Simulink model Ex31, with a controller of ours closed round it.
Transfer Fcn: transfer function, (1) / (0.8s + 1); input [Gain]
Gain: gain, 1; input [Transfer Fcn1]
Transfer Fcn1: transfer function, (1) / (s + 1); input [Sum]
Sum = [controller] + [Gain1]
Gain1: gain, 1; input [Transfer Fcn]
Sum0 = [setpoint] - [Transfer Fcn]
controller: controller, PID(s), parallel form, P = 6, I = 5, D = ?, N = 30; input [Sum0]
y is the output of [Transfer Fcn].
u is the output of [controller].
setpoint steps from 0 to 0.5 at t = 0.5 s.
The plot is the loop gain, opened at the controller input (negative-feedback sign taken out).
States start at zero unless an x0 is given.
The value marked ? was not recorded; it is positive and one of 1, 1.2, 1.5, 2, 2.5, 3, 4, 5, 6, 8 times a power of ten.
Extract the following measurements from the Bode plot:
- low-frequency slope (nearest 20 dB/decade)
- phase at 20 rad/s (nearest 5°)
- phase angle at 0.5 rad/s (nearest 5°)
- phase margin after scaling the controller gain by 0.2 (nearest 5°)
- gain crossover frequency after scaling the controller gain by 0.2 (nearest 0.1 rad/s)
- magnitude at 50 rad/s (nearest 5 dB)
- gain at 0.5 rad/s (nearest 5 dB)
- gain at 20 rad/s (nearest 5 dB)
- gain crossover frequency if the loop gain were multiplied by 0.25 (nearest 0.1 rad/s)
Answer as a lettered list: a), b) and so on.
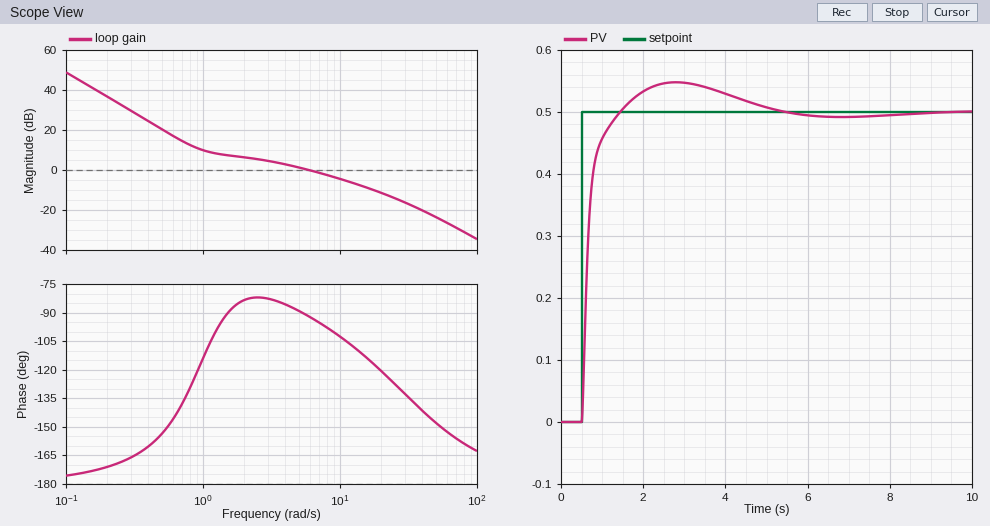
a) -40 dB/decade
b) -120°
c) -155°
d) 45°
e) 0.7 rad/s
f) -25 dB
g) 20 dB
h) -10 dB
i) 0.8 rad/s
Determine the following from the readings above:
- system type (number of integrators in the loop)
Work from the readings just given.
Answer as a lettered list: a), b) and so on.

a) 2
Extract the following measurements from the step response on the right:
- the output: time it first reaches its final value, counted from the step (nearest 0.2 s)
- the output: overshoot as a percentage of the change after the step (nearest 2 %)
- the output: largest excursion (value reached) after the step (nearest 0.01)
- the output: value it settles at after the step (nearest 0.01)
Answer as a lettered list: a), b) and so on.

a) 1.0 s
b) 10 %
c) 0.55
d) 0.50
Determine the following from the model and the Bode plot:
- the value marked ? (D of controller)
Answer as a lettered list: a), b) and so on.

a) 5
